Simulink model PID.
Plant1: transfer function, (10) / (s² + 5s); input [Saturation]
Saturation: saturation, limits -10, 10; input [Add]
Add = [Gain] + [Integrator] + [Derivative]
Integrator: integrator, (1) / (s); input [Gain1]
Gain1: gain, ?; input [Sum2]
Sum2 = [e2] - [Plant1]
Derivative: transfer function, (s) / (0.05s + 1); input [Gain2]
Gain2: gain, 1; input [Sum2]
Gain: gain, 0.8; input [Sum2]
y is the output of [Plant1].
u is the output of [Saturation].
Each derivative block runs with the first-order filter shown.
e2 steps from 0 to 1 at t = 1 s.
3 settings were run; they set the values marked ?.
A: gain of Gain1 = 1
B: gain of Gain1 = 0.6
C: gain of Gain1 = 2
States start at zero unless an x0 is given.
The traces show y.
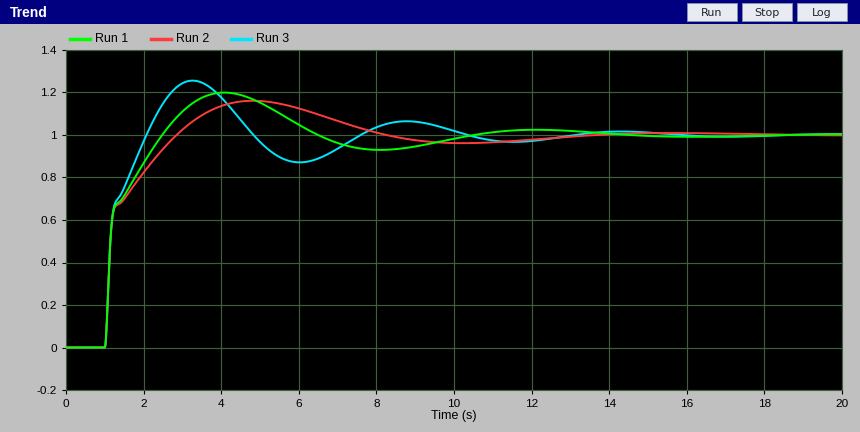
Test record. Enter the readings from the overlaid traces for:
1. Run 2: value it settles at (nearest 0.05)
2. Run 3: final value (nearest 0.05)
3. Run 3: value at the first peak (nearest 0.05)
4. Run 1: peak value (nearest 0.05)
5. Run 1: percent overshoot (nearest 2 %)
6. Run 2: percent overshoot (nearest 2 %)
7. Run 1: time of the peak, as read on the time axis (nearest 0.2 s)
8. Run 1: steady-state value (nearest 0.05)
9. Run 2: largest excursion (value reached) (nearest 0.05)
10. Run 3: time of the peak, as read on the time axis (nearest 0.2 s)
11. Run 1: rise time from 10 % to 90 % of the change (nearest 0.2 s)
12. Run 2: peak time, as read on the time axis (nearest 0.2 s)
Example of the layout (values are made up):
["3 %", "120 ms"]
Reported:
["1.00", "1.00", "1.25", "1.20", "20 %", "16 %", "4.0 s", "1.00", "1.15", "3.2 s", "1.0 s", "4.8 s"]
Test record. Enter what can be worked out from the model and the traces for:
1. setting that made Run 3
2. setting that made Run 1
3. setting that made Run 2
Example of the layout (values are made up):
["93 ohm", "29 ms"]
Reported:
["C", "A", "B"]
